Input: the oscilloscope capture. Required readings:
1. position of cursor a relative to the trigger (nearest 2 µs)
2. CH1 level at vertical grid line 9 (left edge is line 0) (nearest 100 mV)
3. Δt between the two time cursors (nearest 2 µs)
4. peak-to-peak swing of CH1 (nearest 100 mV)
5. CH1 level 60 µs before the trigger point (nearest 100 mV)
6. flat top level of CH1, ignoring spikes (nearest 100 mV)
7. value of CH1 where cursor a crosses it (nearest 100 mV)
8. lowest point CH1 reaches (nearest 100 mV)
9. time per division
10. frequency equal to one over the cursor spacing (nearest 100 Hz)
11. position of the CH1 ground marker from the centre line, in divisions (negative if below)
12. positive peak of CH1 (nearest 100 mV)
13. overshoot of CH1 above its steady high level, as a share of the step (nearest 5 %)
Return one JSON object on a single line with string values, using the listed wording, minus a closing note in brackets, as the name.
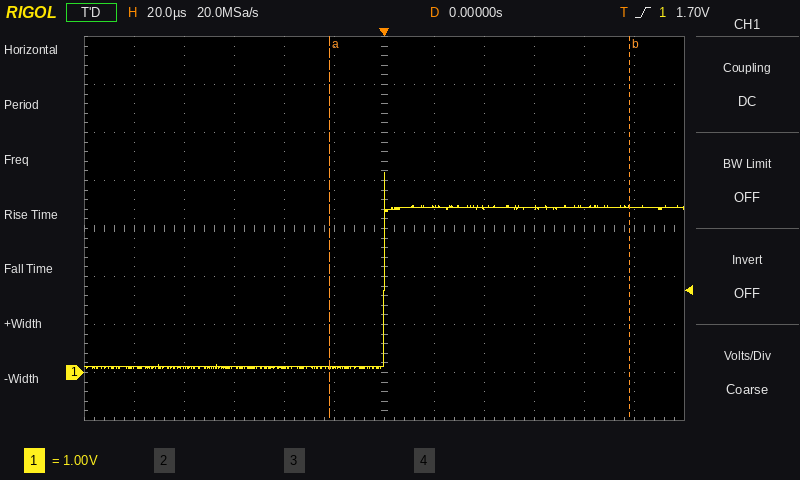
{"position of cursor a relative to the trigger": "-22 µs", "CH1 level at vertical grid line 9 (left edge is line 0)": "3.4 V", "Δt between the two time cursors": "120 µs", "peak-to-peak swing of CH1": "4.1 V", "CH1 level 60 µs before the trigger point": "100 mV", "flat top level of CH1, ignoring spikes": "3.4 V", "value of CH1 where cursor a crosses it": "100 mV", "lowest point CH1 reaches": "100 mV", "time per division": "20 µs", "frequency equal to one over the cursor spacing": "8.3 kHz", "position of the CH1 ground marker from the centre line, in divisions": "-3.0 div", "positive peak of CH1": "4.2 V", "overshoot of CH1 above its steady high level, as a share of the step": "20 %"}
